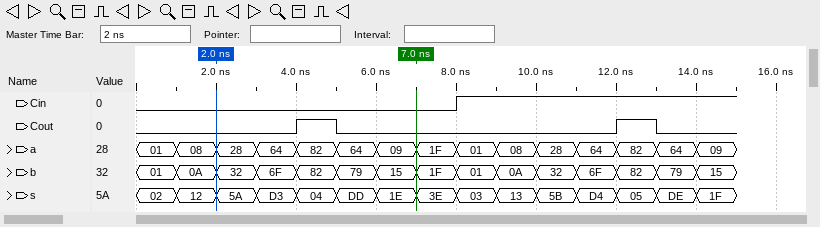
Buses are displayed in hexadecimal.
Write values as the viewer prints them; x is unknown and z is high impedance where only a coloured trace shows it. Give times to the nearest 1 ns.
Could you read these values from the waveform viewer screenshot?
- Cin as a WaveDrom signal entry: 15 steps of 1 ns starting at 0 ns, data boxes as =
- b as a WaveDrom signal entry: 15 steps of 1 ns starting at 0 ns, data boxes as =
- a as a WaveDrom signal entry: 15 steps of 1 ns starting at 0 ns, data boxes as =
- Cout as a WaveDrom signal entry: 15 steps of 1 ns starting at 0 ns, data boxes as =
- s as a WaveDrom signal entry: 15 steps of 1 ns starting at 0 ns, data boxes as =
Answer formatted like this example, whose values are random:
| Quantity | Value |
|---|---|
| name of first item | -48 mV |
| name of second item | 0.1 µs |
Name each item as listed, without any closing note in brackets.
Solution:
| Quantity | Value |
|---|---|
| Cin as a WaveDrom signal entry: 15 steps of 1 ns starting at 0 ns, data boxes as = | {name: 'Cin', wave: '0.......1......'} |
| b as a WaveDrom signal entry: 15 steps of 1 ns starting at 0 ns, data boxes as = | {name: 'b', wave: '===============', data: '01 0A 32 6F 82 79 15 1F 01 0A 32 6F 82 79 15'} |
| a as a WaveDrom signal entry: 15 steps of 1 ns starting at 0 ns, data boxes as = | {name: 'a', wave: '===============', data: '01 08 28 64 82 64 09 1F 01 08 28 64 82 64 09'} |
| Cout as a WaveDrom signal entry: 15 steps of 1 ns starting at 0 ns, data boxes as = | {name: 'Cout', wave: '0...10......10.'} |
| s as a WaveDrom signal entry: 15 steps of 1 ns starting at 0 ns, data boxes as = | {name: 's', wave: '===============', data: '02 12 5A D3 04 DD 1E 3E 03 13 5B D4 05 DE 1F'} |
